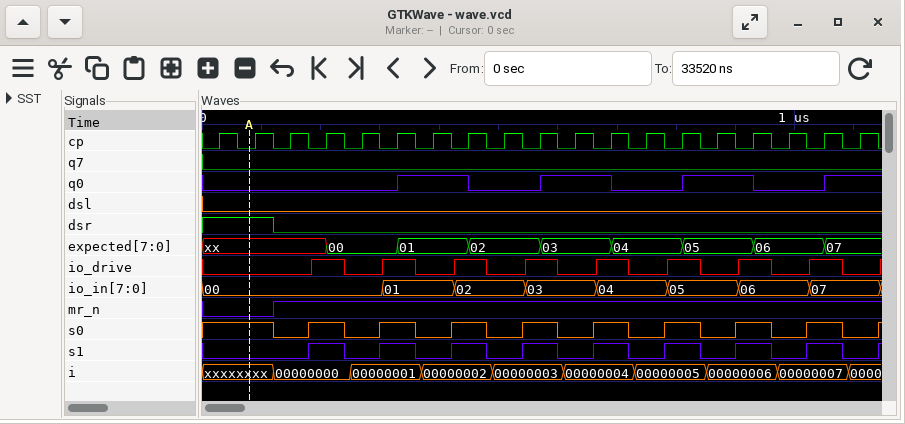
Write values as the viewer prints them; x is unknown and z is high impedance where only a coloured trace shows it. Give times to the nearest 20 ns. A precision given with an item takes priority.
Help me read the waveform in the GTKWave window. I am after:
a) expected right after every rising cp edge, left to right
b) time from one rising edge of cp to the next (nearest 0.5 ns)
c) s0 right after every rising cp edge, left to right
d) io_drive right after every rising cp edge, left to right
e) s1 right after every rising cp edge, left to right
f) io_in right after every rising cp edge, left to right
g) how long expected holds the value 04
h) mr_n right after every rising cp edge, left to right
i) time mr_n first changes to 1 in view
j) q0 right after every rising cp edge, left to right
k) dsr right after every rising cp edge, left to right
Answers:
xx, xx, xx, 00, 00, 01, 01, 02, 02, 03, 03, 04, 04, 05, 05, 06, 06, 07, 07
60 ns
1 1 0 1 0 1 0 1 0 1 0 1 0 1 0 1 0 1 0
0 0 0 1 0 1 0 1 0 1 0 1 0 1 0 1 0 1 0
0 0 0 1 0 1 0 1 0 1 0 1 0 1 0 1 0 1 0
00, 00, 00, 00, 00, 01, 01, 02, 02, 03, 03, 04, 04, 05, 05, 06, 06, 07, 07
120 ns
0 0 1 1 1 1 1 1 1 1 1 1 1 1 1 1 1 1 1
120 ns
0 0 0 0 0 1 1 0 0 1 1 0 0 1 1 0 0 1 1
1 1 0 0 0 0 0 0 0 0 0 0 0 0 0 0 0 0 0
